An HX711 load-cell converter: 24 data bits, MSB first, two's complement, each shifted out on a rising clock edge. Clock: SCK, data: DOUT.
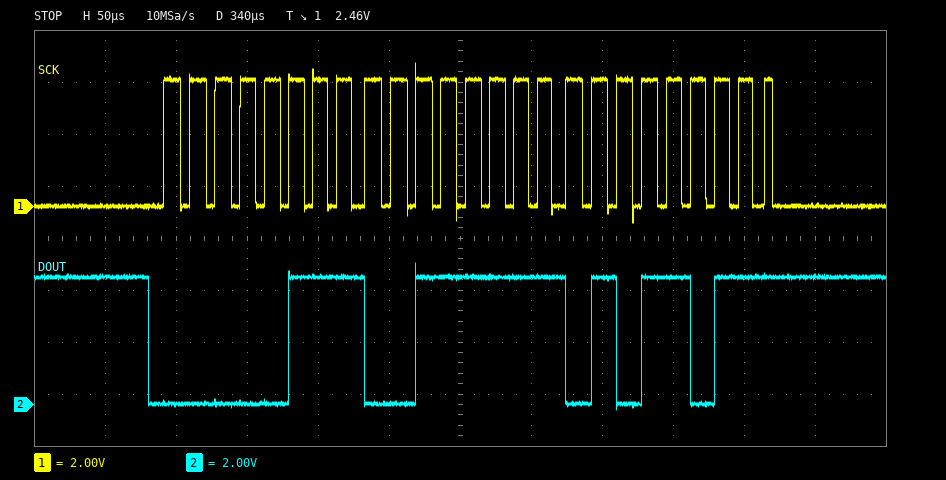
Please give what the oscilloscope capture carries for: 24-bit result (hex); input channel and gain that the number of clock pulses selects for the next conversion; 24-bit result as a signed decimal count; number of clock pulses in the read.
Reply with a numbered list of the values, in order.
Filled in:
1. 0x073F5B
2. channel A, gain 128
3. 474971
4. 25
